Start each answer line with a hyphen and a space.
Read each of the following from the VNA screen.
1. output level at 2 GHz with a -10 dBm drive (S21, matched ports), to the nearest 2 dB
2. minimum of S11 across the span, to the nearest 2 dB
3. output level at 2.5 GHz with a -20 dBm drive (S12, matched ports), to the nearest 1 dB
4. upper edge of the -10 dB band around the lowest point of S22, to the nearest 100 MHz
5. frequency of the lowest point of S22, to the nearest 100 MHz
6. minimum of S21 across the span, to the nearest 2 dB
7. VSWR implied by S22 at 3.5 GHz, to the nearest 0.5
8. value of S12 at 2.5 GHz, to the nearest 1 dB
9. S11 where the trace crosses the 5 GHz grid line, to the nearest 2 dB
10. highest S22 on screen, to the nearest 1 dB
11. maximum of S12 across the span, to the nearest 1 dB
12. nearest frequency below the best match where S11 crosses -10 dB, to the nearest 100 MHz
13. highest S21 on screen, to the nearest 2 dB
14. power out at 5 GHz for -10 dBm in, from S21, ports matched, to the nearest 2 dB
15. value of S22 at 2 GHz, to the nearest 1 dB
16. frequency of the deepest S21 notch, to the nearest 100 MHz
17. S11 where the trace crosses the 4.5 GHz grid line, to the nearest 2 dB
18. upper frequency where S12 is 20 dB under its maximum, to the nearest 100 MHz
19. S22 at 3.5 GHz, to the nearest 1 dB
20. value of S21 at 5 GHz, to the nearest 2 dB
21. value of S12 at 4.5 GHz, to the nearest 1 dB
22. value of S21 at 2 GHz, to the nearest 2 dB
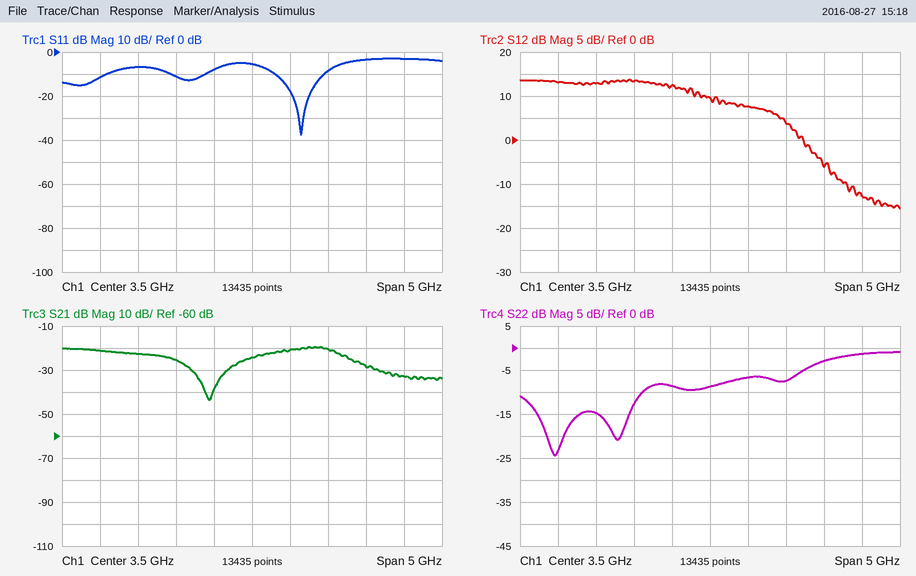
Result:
- -32 dBm
- -38 dB
- -7 dBm
- 2.6 GHz
- 1.5 GHz
- -44 dB
- 2.0
- 13 dB
- -4 dB
- -1 dB
- 14 dB
- 3.8 GHz
- -20 dB
- -38 dBm
- -15 dB
- 2.9 GHz
- -8 dB
- 5.1 GHz
- -9 dB
- -28 dB
- 4 dB
- -22 dB
